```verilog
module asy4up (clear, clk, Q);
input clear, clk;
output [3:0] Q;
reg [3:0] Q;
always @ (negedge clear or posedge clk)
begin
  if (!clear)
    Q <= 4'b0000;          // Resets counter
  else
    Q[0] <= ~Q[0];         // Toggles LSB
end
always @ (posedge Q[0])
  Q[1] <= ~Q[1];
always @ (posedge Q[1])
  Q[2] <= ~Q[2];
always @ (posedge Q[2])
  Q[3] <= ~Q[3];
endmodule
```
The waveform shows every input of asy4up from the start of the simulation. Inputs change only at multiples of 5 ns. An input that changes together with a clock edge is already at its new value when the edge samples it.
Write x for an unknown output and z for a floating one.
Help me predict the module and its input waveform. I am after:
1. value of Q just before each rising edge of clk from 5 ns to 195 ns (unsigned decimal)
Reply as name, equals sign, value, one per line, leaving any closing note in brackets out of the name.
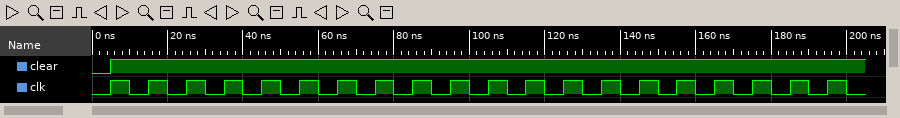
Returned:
value of Q just before each rising edge of clk from 5 ns to 195 ns = 0, 15, 14, 13, 12, 11, 10, 9, 8, 7, 6, 5, 4, 3, 2, 1, 0, 15, 14, 13
